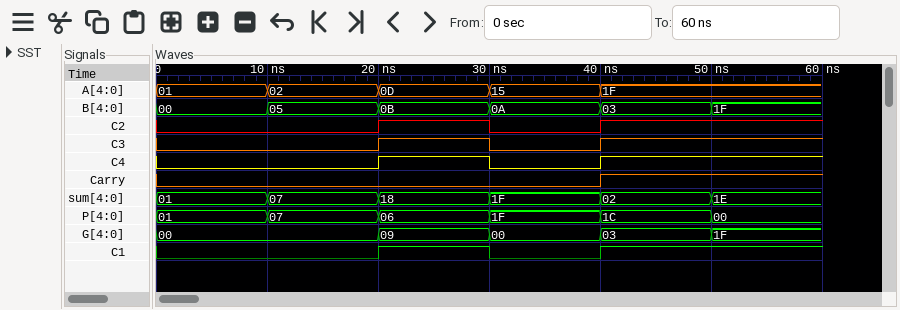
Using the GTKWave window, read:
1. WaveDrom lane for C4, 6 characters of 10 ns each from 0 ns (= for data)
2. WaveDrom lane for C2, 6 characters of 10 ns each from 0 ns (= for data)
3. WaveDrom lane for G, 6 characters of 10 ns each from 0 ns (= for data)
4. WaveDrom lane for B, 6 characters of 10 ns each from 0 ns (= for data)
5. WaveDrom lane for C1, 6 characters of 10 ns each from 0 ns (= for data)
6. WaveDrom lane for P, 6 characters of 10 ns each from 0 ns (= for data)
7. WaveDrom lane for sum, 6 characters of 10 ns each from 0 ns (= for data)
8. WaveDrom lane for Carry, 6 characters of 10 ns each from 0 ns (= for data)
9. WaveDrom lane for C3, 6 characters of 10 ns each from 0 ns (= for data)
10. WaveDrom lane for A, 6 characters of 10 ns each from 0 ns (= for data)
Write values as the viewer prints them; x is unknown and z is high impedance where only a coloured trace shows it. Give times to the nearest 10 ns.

{name: 'C4', wave: '0.101.'}
{name: 'C2', wave: '0.101.'}
{name: 'G', wave: '=.====', data: '00 09 00 03 1F'}
{name: 'B', wave: '======', data: '00 05 0B 0A 03 1F'}
{name: 'C1', wave: '0.101.'}
{name: 'P', wave: '======', data: '01 07 06 1F 1C 00'}
{name: 'sum', wave: '======', data: '01 07 18 1F 02 1E'}
{name: 'Carry', wave: '0...1.'}
{name: 'C3', wave: '0.101.'}
{name: 'A', wave: '=====.', data: '01 02 0D 15 1F'}
